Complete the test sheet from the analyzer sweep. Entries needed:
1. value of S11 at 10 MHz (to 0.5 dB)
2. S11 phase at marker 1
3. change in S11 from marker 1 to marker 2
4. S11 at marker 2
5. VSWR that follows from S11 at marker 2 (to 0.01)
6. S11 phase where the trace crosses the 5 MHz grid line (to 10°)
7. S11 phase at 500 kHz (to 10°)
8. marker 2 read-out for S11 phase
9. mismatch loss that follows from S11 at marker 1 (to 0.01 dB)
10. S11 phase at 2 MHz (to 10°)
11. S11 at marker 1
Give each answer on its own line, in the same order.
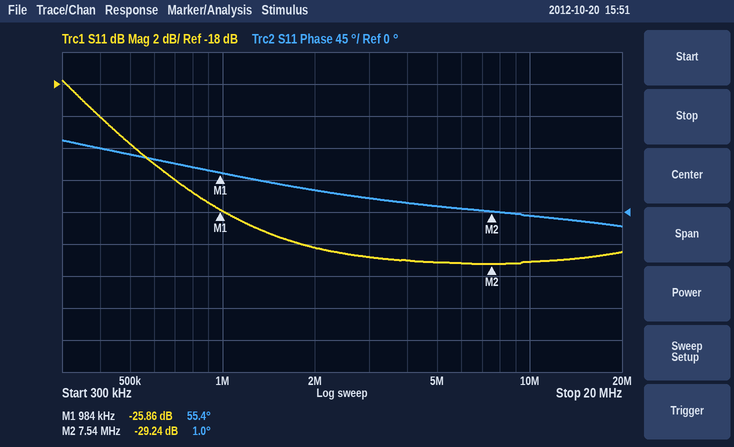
-29.0 dB
55.4°
-3.38 dB
-29.24 dB
1.07
10°
80°
1.0°
0.01 dB
30°
-25.86 dB
